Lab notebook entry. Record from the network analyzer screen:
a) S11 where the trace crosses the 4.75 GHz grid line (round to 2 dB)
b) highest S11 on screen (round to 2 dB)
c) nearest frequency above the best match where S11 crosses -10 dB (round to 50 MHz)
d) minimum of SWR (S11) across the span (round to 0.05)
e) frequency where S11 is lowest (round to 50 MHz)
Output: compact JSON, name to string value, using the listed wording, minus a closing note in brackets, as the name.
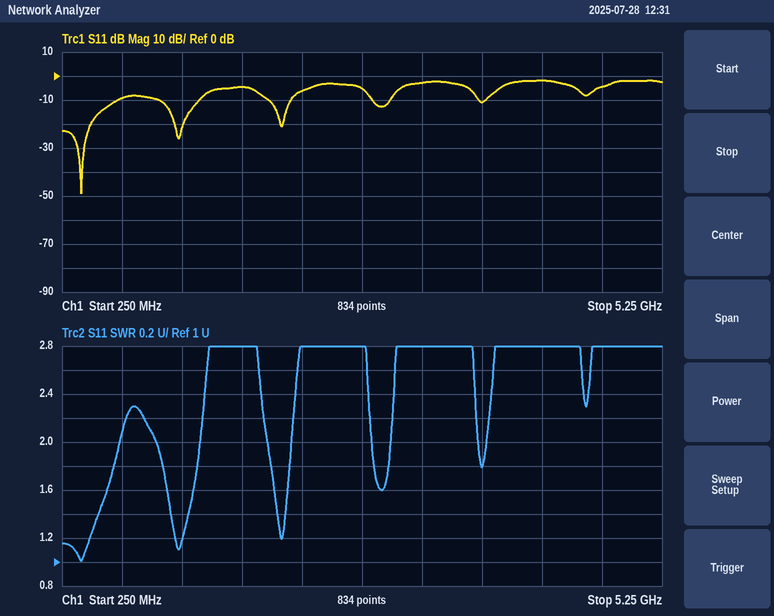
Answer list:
{"S11 where the trace crosses the 4.75 GHz grid line": "-4 dB", "highest S11 on screen": "-2 dB", "nearest frequency above the best match where S11 crosses -10 dB": "700 MHz", "minimum of SWR (S11) across the span": "1.00", "frequency where S11 is lowest": "400 MHz"}
